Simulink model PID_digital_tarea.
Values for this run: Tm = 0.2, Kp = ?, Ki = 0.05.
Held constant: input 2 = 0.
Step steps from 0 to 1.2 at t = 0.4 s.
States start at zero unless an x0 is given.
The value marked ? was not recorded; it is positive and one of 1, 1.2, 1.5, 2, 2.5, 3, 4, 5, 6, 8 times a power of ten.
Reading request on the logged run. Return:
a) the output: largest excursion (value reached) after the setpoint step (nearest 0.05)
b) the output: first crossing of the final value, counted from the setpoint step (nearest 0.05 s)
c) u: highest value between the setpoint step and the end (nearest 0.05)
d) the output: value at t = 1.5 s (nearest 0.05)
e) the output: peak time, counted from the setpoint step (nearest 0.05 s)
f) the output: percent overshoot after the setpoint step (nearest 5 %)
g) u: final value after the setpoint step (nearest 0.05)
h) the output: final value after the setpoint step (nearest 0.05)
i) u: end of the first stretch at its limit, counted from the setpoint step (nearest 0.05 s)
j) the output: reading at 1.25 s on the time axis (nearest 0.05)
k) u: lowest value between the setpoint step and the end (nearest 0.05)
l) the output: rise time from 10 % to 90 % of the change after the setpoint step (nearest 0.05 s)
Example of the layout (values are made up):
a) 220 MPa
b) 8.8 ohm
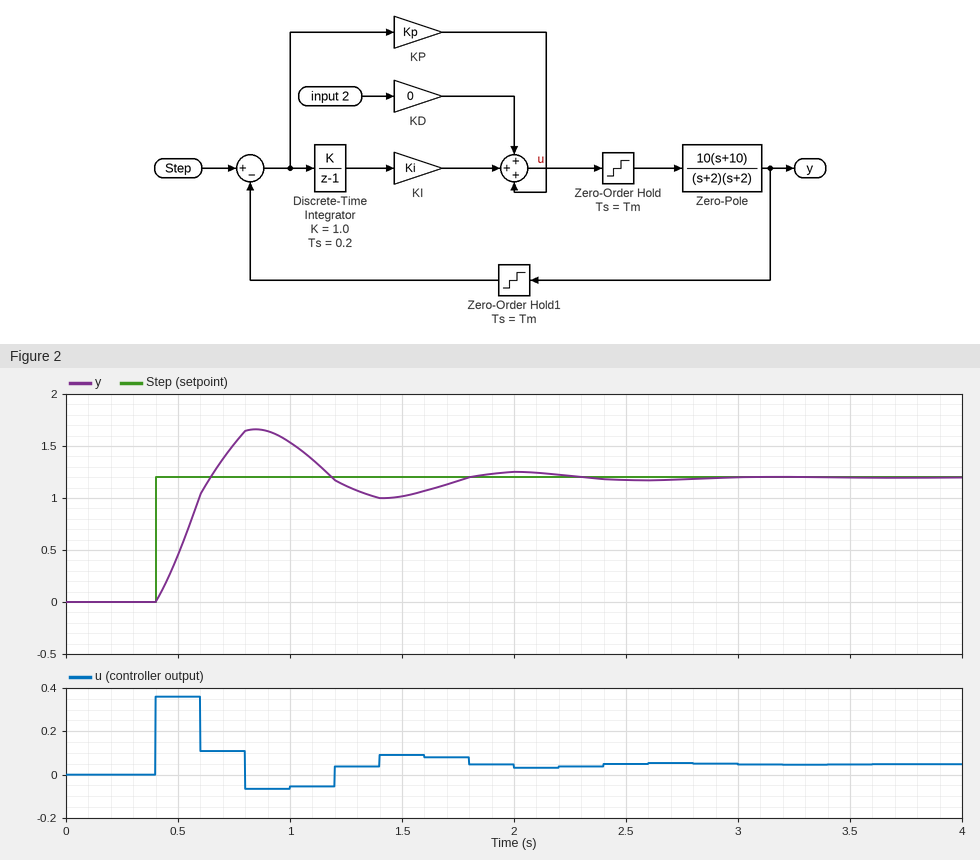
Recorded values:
a) 1.65
b) 0.25 s
c) 0.35
d) 1.00
e) 0.45 s
f) 40 %
g) 0.05
h) 1.20
i) 0.20 s
j) 1.10
k) -0.05
l) 0.20 s
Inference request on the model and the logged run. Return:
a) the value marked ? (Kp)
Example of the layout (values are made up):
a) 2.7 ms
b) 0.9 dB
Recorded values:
a) 0.3
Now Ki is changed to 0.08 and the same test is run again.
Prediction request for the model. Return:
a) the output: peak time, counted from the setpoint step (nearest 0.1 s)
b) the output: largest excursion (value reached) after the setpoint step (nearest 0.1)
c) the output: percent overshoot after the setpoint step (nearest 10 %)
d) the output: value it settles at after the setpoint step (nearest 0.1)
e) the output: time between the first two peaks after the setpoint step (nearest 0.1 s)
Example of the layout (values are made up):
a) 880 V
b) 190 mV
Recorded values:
a) 0.5 s
b) 1.8
c) 50 %
d) 1.2
e) 1.2 s
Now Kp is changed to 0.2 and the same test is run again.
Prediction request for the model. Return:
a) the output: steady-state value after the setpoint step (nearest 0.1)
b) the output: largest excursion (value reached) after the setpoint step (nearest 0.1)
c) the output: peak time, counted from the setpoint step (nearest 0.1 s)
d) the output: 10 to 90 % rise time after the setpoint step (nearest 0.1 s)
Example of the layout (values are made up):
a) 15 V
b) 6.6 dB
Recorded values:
a) 1.2
b) 1.6
c) 0.6 s
d) 0.3 s
